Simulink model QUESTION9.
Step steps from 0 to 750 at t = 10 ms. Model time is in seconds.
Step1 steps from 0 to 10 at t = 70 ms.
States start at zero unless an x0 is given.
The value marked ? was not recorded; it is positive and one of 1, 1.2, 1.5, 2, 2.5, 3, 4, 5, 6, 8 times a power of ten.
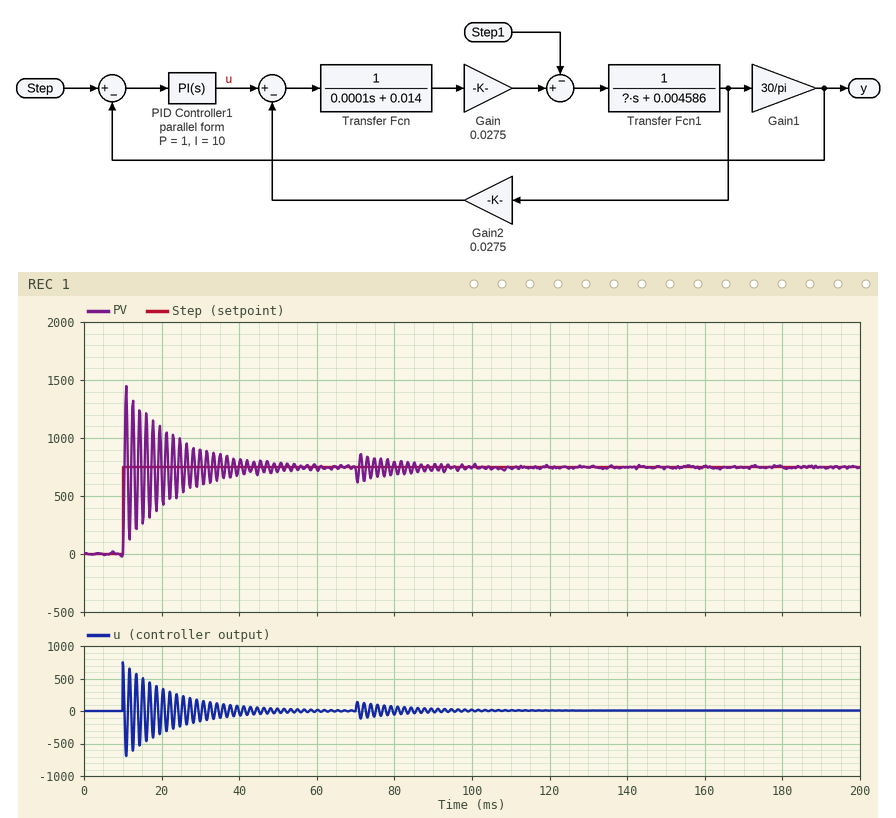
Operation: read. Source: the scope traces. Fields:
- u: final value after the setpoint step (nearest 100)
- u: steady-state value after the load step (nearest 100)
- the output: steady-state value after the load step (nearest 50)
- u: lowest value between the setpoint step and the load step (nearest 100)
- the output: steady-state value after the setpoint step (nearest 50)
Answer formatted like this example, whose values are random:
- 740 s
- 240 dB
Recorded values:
- 0
- 0
- 750
- -700
- 750
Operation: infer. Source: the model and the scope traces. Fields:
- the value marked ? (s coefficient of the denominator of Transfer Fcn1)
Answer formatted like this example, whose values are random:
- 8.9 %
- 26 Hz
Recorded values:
- 0.0002
